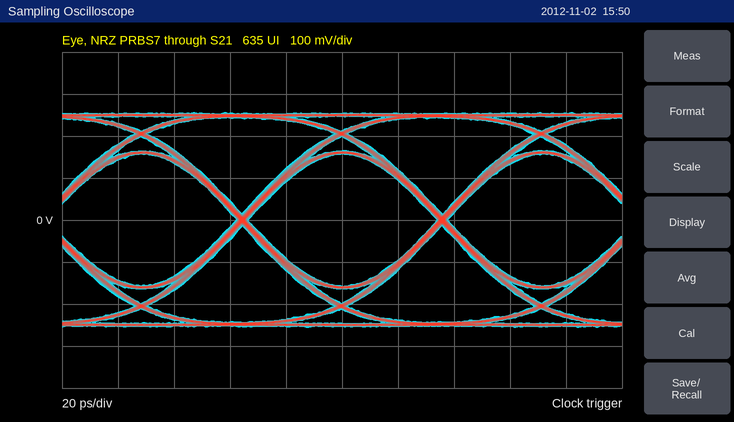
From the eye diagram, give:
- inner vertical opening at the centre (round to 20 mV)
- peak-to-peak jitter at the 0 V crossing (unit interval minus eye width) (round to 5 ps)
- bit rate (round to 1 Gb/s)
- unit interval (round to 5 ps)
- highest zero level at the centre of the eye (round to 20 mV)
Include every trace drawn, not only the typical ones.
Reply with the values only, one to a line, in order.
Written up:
320 mV
5 ps
14 Gb/s
70 ps
-160 mV
